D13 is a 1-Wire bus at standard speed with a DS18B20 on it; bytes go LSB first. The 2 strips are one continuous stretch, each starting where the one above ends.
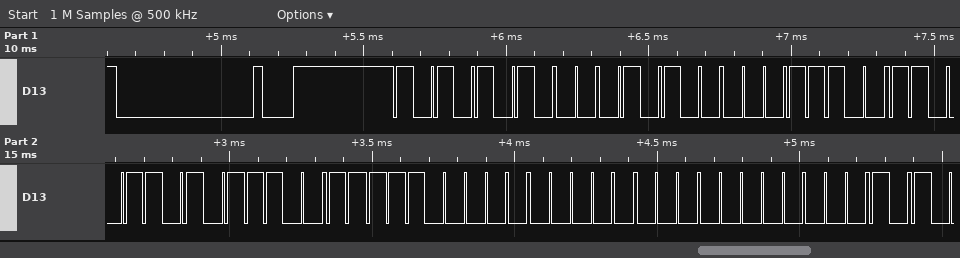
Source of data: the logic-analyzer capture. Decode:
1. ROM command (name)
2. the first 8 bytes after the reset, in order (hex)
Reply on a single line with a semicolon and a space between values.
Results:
Match ROM; 55 28 38 B3 CE 07 00 00
